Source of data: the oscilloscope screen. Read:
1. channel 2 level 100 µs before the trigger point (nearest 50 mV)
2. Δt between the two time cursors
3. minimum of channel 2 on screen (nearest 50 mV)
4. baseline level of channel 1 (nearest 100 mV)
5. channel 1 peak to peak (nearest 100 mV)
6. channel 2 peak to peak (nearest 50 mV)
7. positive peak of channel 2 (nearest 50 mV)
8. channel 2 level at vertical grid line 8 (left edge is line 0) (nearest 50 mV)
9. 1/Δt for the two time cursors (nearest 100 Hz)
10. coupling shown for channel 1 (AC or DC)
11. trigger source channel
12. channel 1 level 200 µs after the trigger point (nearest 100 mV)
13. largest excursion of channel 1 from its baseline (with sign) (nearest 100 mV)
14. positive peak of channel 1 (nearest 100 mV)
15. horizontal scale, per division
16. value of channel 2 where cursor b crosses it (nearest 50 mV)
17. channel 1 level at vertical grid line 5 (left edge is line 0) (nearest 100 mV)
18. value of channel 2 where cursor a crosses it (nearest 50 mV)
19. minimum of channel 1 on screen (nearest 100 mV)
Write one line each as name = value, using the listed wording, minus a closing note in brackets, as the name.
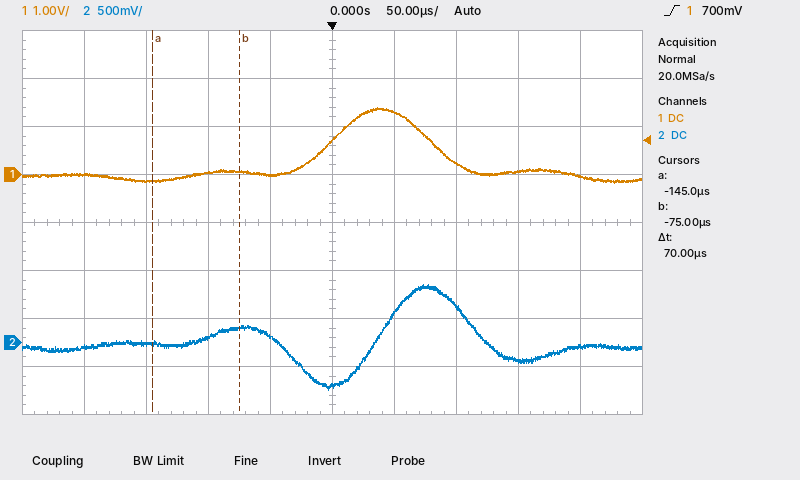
channel 2 level 100 µs before the trigger point = 50 mV
Δt between the two time cursors = 70 µs
minimum of channel 2 on screen = -500 mV
baseline level of channel 1 = 0.0 V
channel 1 peak to peak = 1.6 V
channel 2 peak to peak = 1.10 V
positive peak of channel 2 = 600 mV
channel 2 level at vertical grid line 8 (left edge is line 0) = -200 mV
1/Δt for the two time cursors = 14.3 kHz
coupling shown for channel 1 = DC
trigger source channel = channel 1
channel 1 level 200 µs after the trigger point = 0.0 V
largest excursion of channel 1 from its baseline (with sign) = +1.4 V
positive peak of channel 1 = 1.4 V
horizontal scale, per division = 50 µs
value of channel 2 where cursor b crosses it = 150 mV
channel 1 level at vertical grid line 5 (left edge is line 0) = 700 mV
value of channel 2 where cursor a crosses it = 0 mV
minimum of channel 1 on screen = -200 mV
